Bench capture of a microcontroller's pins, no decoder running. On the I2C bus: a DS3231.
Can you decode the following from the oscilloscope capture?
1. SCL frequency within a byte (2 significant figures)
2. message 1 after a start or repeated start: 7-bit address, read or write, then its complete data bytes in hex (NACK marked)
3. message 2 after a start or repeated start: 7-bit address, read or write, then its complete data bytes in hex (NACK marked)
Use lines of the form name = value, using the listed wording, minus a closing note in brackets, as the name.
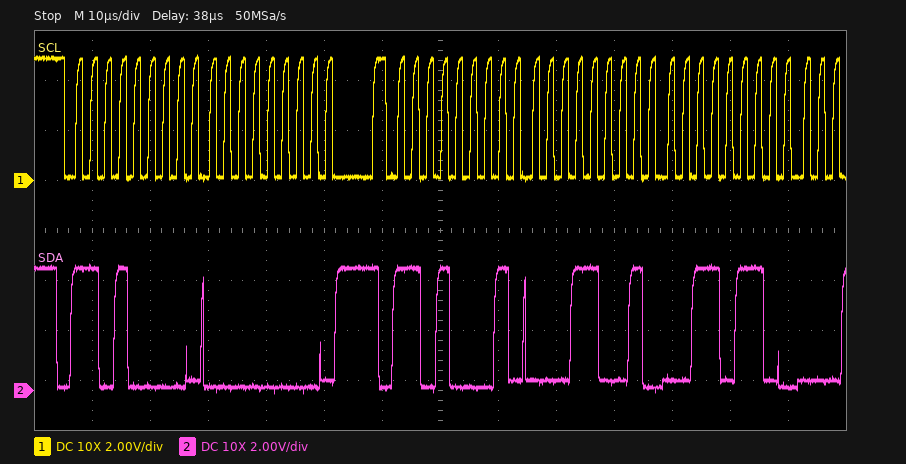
SCL frequency within a byte = 400 kHz
message 1 after a start or repeated start: 7-bit address, read or write, then its complete data bytes in hex = 0x68 write: 00
message 2 after a start or repeated start: 7-bit address, read or write, then its complete data bytes in hex = 0x68 read: 19 36
